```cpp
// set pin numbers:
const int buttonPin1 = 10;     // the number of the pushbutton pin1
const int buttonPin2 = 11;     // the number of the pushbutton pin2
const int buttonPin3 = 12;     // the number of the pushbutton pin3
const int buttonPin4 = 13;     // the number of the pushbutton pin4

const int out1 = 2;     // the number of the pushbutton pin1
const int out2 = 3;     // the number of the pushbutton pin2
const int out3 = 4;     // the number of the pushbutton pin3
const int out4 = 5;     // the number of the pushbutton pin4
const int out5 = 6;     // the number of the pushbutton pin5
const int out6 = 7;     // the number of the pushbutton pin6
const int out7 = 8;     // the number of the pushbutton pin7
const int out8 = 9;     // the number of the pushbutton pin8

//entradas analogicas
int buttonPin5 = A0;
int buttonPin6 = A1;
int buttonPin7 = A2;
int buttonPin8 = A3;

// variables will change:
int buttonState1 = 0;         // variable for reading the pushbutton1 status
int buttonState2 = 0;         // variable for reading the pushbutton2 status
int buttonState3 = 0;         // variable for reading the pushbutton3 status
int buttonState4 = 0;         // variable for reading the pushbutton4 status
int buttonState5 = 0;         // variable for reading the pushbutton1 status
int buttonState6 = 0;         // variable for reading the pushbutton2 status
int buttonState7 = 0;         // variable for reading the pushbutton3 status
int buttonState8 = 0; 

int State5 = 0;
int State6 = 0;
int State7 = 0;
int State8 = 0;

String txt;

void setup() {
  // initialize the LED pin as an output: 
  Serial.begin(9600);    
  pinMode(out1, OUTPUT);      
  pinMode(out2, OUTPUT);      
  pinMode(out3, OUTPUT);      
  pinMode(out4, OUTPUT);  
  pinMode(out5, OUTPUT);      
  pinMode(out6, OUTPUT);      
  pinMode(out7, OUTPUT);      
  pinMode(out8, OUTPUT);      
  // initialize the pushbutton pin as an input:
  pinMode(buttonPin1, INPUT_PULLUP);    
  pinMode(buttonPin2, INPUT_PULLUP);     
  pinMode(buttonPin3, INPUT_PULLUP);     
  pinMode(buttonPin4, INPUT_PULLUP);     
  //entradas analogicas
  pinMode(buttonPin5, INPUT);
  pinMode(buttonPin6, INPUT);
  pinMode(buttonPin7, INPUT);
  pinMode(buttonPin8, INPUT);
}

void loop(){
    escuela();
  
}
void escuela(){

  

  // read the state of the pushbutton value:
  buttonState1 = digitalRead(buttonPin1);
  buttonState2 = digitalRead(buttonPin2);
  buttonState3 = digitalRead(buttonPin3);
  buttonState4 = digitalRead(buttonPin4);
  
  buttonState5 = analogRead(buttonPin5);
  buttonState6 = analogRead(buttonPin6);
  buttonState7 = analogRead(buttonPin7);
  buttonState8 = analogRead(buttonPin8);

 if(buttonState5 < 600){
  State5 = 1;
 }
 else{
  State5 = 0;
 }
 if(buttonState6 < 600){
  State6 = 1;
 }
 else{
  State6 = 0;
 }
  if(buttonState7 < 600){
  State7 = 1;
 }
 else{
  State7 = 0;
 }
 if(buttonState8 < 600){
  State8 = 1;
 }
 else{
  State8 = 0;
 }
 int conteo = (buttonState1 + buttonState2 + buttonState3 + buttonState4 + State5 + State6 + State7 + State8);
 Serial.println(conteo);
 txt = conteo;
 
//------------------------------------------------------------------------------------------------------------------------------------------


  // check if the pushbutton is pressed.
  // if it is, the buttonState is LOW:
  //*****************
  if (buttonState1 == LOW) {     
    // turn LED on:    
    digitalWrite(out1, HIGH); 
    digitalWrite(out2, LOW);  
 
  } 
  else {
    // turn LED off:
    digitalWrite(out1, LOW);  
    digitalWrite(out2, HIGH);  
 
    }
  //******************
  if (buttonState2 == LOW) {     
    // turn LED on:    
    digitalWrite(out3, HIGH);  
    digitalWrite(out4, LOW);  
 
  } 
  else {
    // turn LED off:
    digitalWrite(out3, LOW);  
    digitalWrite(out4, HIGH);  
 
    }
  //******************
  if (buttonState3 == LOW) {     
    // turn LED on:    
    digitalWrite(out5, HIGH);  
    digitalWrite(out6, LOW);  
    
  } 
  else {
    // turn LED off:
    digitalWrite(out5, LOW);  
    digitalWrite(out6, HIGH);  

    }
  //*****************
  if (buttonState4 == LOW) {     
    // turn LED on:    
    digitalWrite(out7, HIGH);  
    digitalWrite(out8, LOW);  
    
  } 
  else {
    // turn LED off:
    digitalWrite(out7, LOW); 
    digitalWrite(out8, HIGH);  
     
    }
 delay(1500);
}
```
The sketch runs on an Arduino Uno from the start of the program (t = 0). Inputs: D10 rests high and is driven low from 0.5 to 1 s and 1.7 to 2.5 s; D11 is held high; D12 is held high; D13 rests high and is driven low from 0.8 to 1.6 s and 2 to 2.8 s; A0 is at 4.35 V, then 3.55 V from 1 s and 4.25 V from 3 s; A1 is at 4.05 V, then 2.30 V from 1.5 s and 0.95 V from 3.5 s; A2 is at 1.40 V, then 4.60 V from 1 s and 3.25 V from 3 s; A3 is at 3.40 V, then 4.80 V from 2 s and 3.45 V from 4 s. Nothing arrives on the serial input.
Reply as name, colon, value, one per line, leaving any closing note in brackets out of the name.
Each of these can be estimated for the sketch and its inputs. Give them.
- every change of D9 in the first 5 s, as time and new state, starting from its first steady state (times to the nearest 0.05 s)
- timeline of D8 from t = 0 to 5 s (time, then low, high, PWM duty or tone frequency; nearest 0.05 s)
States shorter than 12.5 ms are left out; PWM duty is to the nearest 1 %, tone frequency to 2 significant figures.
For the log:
every change of D9 in the first 5 s, as time and new state, starting from its first steady state: 0 s high; 1.5 s low; 3 s high
timeline of D8 from t = 0 to 5 s: 0 s low; 1.5 s high; 3 s low
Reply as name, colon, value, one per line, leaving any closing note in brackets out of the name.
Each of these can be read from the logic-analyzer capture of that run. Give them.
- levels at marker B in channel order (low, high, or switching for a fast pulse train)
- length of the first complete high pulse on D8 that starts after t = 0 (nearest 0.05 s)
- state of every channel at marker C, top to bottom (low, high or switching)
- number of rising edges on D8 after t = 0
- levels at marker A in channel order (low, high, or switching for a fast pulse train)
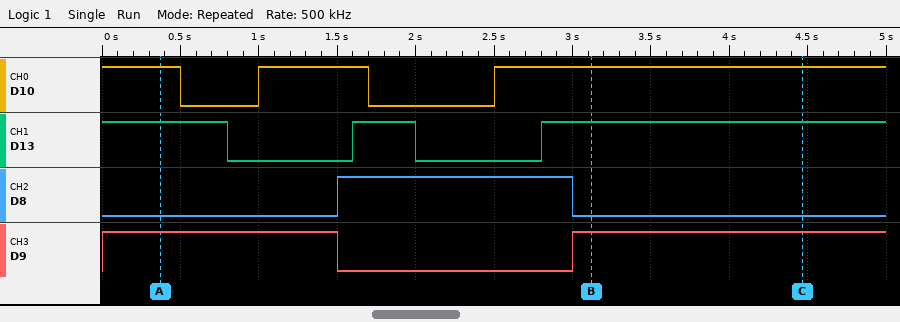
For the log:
levels at marker B in channel order: D10 high, D13 high, D8 low, D9 high
length of the first complete high pulse on D8 that starts after t = 0: 1.50 s
state of every channel at marker C, top to bottom: D10 high, D13 high, D8 low, D9 high
number of rising edges on D8 after t = 0: 1
levels at marker A in channel order: D10 high, D13 high, D8 low, D9 high
